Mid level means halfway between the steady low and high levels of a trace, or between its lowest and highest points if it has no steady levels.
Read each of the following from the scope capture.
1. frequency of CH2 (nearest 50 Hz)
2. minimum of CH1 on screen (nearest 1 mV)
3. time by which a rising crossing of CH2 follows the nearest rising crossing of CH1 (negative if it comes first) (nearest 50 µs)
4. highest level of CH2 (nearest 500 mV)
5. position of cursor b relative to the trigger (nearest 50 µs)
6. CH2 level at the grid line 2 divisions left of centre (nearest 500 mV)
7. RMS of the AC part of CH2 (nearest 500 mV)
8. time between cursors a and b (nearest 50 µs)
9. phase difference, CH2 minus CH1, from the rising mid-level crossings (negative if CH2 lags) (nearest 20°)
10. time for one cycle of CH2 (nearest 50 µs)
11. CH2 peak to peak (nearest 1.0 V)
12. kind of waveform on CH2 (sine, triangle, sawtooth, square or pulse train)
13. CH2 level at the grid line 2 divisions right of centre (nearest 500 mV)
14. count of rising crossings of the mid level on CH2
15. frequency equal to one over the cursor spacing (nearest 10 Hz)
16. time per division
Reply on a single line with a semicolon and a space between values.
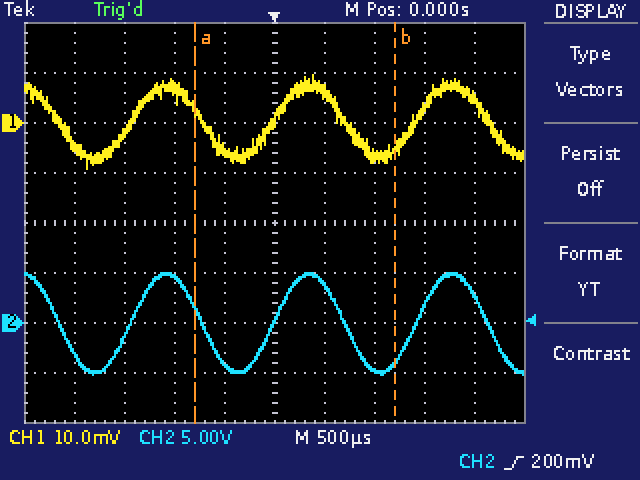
700 Hz; -9 mV; 0 µs; 5.0 V; +1.20 ms; 4.5 V; 3.5 V; 2.00 ms; 0°; 1.45 ms; 10.0 V; sine; -4.5 V; 3; 500 Hz; 500 µs
